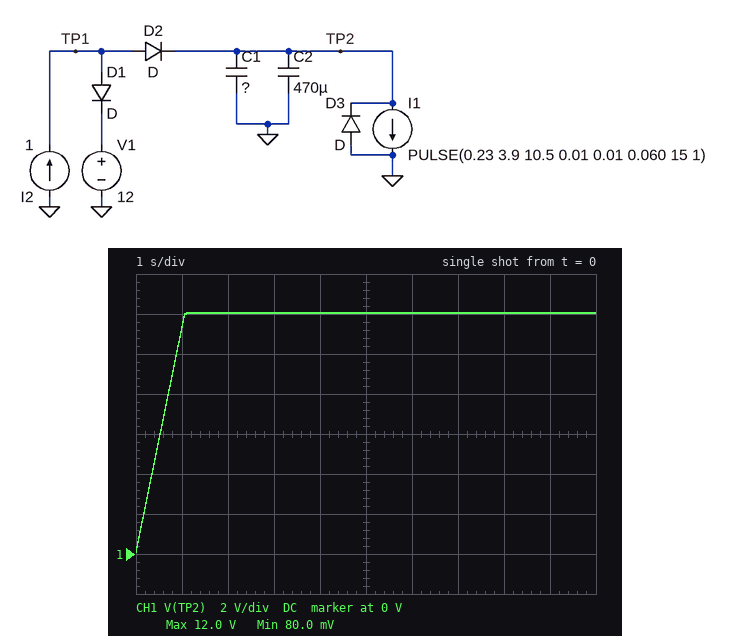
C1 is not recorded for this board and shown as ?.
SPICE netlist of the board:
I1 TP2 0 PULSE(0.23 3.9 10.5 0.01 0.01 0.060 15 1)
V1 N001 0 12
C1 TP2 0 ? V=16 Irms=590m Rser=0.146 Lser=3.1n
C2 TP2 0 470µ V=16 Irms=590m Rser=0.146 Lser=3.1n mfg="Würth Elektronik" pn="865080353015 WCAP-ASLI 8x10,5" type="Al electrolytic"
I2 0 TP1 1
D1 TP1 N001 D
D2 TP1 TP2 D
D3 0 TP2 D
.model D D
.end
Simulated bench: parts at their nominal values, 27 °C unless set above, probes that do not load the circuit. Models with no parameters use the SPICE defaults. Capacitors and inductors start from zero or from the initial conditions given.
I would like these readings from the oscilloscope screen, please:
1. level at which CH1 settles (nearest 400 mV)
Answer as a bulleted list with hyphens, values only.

- 12.0 V
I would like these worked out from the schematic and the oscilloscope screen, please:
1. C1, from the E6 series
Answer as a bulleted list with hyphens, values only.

- 68 mF
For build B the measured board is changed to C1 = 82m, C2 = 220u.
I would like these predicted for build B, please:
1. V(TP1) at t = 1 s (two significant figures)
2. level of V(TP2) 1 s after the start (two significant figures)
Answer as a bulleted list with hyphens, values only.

- 10 V
- 9.5 V
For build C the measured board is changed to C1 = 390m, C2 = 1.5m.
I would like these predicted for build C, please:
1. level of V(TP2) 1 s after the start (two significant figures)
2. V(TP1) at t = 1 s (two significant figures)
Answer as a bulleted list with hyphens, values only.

- 2.1 V
- 2.9 V
